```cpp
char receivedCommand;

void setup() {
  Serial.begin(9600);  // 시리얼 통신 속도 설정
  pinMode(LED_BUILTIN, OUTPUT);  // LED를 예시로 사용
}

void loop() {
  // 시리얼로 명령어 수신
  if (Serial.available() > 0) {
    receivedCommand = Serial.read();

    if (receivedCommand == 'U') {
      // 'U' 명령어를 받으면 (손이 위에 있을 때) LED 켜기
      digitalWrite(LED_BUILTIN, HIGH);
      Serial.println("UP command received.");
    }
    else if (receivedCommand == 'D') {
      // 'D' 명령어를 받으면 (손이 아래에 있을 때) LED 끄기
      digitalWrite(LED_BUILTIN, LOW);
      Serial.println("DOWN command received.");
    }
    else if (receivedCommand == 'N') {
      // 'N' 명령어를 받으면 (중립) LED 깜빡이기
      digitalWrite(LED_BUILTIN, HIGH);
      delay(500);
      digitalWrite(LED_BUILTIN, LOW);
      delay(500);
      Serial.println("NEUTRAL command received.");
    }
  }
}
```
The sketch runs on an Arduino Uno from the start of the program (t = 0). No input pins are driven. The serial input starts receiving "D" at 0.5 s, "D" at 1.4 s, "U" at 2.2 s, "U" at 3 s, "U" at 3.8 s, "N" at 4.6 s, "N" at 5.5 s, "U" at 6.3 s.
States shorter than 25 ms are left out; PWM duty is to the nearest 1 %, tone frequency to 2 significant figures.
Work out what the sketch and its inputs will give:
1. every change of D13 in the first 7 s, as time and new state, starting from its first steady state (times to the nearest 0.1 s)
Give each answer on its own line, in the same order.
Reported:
0 s low; 2.2 s high; 5.1 s low; 5.6 s high; 6.1 s low; 6.6 s high
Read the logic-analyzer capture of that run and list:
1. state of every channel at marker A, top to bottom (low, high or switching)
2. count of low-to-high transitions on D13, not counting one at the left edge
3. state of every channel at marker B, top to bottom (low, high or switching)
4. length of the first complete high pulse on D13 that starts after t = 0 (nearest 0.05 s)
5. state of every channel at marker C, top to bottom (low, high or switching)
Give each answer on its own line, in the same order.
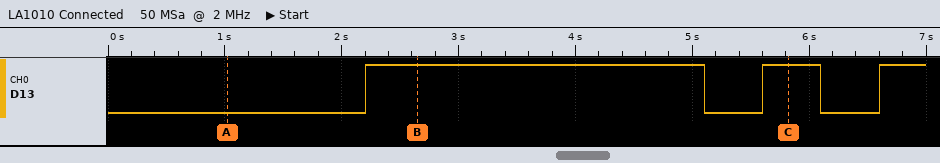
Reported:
D13 low
3
D13 high
2.90 s
D13 high
